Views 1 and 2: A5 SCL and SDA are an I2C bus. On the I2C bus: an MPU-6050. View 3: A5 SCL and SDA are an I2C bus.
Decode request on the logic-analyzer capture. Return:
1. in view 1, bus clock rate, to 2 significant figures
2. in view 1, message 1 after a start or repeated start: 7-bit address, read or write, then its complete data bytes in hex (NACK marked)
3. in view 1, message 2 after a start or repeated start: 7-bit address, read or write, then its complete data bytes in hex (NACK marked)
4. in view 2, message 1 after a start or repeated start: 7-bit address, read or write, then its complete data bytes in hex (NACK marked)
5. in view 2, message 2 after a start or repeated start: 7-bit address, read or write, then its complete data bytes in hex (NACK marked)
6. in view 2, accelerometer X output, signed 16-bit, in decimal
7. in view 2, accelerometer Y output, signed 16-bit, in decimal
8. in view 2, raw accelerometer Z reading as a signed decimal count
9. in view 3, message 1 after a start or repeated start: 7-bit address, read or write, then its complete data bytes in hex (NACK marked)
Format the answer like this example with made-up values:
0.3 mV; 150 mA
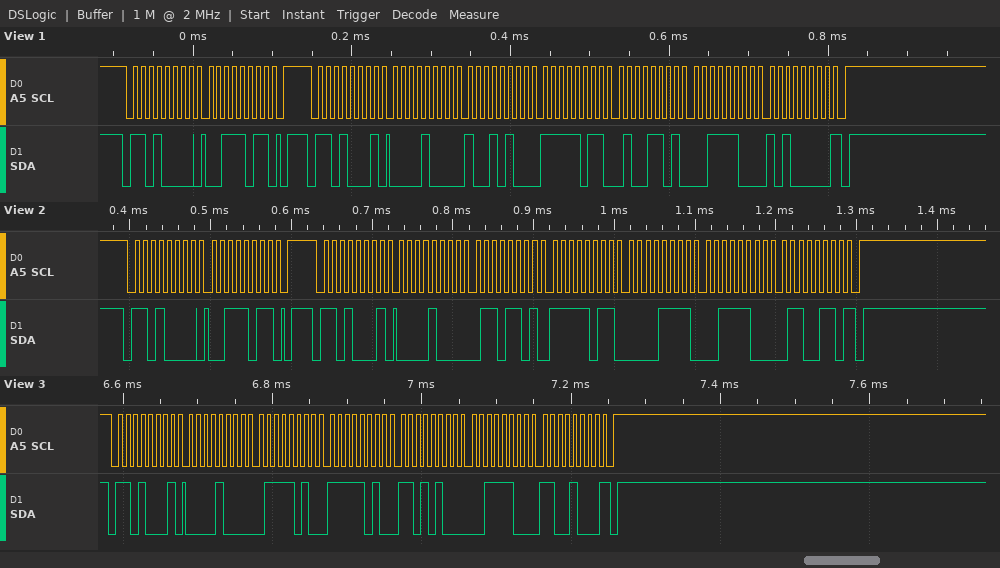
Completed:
100 kHz; 0x68 write: 3B; 0x68 read: 08 94 FB 4D 3C A0 NACK; 0x68 write: 3B; 0x68 read: 08 6D FB 0F 3C 66 NACK; 2157; -1265; 15462; 0x68 read: 08 7A FA D4 3C C8 NACK
